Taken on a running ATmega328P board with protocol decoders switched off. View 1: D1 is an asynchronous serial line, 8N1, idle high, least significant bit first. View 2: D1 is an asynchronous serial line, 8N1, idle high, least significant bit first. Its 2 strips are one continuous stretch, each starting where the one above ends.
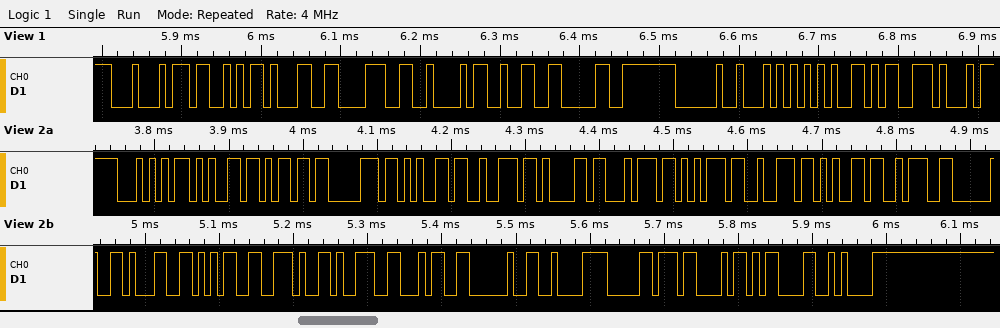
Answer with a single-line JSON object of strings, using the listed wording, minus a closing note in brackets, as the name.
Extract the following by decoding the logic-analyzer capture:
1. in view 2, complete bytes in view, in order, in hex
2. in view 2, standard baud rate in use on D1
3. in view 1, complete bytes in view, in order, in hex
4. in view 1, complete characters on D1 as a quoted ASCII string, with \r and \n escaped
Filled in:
{"in view 2, complete bytes in view, in order, in hex": "54 65 6D 70 65 72 61 74 75 72 65 3A 20 31 35 2E 39 34 20 C2 B0 43 0D 0A", "in view 2, standard baud rate in use on D1": "115200 baud", "in view 1, complete bytes in view, in order, in hex": "44 53 31 38 42 32 30 20 54 65 73", "in view 1, complete characters on D1 as a quoted ASCII string, with \\r and \\n escaped": "\"DS18B20 Tes\""}
